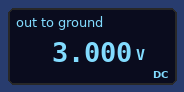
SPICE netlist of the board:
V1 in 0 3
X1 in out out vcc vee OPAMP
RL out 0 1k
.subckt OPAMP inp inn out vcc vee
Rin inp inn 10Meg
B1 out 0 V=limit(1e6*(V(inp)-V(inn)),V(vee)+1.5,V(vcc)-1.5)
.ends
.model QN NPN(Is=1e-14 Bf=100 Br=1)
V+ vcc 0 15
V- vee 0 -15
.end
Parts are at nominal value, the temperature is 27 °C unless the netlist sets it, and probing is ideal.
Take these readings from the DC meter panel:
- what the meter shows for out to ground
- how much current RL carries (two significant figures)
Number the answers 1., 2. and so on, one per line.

1. 3.000 V
2. 3.0 mA
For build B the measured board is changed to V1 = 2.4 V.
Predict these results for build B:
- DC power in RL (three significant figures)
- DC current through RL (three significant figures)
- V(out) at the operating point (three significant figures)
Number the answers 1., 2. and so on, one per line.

1. 5.76 mW
2. 2.40 mA
3. 2.40 V
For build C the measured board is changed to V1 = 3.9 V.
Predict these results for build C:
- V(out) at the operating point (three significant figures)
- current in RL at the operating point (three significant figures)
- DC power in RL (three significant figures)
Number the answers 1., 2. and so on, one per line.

1. 3.90 V
2. 3.90 mA
3. 15.2 mW
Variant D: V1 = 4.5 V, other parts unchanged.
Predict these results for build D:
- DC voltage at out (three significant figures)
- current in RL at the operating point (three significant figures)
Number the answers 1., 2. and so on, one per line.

1. 4.50 V
2. 4.50 mA
